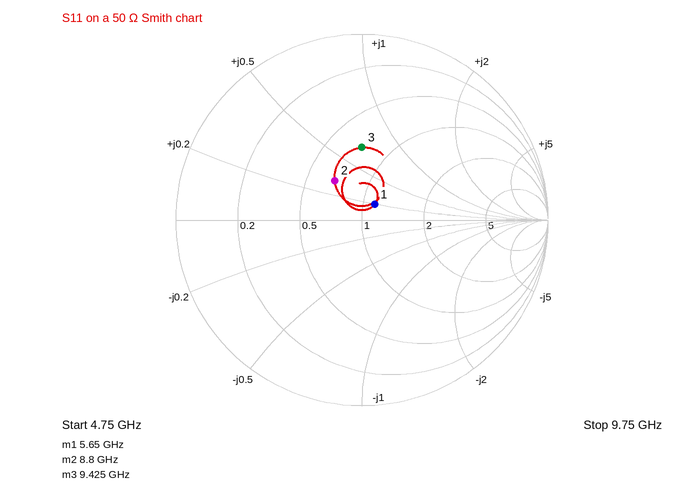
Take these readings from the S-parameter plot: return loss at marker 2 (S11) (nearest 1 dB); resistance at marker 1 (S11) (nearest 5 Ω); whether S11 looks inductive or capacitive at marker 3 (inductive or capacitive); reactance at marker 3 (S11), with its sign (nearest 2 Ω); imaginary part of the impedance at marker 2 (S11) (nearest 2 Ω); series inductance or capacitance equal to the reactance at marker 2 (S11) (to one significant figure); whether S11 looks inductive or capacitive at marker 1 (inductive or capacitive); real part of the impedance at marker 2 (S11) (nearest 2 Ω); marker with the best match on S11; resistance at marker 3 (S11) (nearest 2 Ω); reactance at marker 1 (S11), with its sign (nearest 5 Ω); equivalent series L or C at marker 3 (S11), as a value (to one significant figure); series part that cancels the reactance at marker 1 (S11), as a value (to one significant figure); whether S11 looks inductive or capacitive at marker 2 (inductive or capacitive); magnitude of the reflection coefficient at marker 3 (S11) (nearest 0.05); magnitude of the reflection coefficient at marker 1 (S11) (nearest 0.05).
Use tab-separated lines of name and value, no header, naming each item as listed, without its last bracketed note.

return loss at marker 2 (S11)	12 dB
resistance at marker 1 (S11)	55 Ω
whether S11 looks inductive or capacitive at marker 3	inductive
reactance at marker 3 (S11), with its sign	+34 Ω
imaginary part of the impedance at marker 2 (S11)	+16 Ω
series inductance or capacitance equal to the reactance at marker 2 (S11)	300 pH
whether S11 looks inductive or capacitive at marker 1	inductive
real part of the impedance at marker 2 (S11)	34 Ω
marker with the best match on S11	marker 1
resistance at marker 3 (S11)	36 Ω
reactance at marker 1 (S11), with its sign	+10 Ω
equivalent series L or C at marker 3 (S11), as a value	600 pH
series part that cancels the reactance at marker 1 (S11), as a value	3 pF
whether S11 looks inductive or capacitive at marker 2	inductive
magnitude of the reflection coefficient at marker 3 (S11)	0.40
magnitude of the reflection coefficient at marker 1 (S11)	0.10
